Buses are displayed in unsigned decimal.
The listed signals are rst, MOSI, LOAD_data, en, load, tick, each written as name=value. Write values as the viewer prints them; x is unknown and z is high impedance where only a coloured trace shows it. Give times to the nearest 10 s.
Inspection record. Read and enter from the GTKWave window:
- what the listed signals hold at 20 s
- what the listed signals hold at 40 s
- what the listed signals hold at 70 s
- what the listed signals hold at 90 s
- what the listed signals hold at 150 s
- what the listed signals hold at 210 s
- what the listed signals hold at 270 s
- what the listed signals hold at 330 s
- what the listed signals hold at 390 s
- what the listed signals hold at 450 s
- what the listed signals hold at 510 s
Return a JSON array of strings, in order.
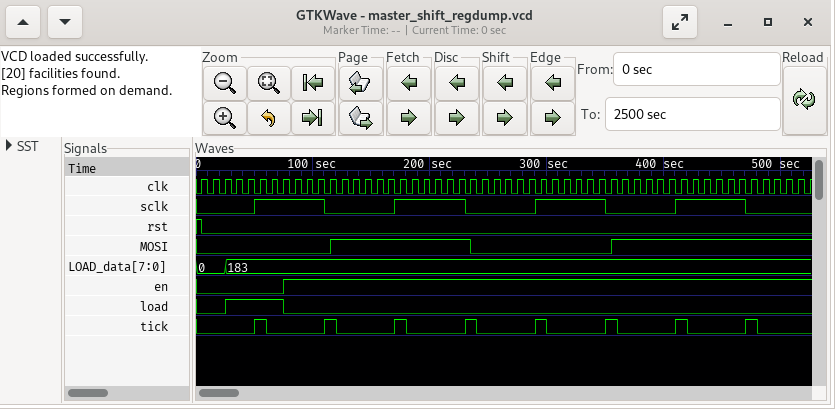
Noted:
["rst=0, MOSI=0, LOAD_data=0, en=0, load=0, tick=0", "rst=0, MOSI=0, LOAD_data=183, en=0, load=1, tick=0", "rst=0, MOSI=0, LOAD_data=183, en=0, load=1, tick=0", "rst=0, MOSI=0, LOAD_data=183, en=1, load=0, tick=0", "rst=0, MOSI=1, LOAD_data=183, en=1, load=0, tick=0", "rst=0, MOSI=1, LOAD_data=183, en=1, load=0, tick=0", "rst=0, MOSI=0, LOAD_data=183, en=1, load=0, tick=0", "rst=0, MOSI=0, LOAD_data=183, en=1, load=0, tick=0", "rst=0, MOSI=1, LOAD_data=183, en=1, load=0, tick=0", "rst=0, MOSI=1, LOAD_data=183, en=1, load=0, tick=0", "rst=0, MOSI=1, LOAD_data=183, en=1, load=0, tick=0"]
